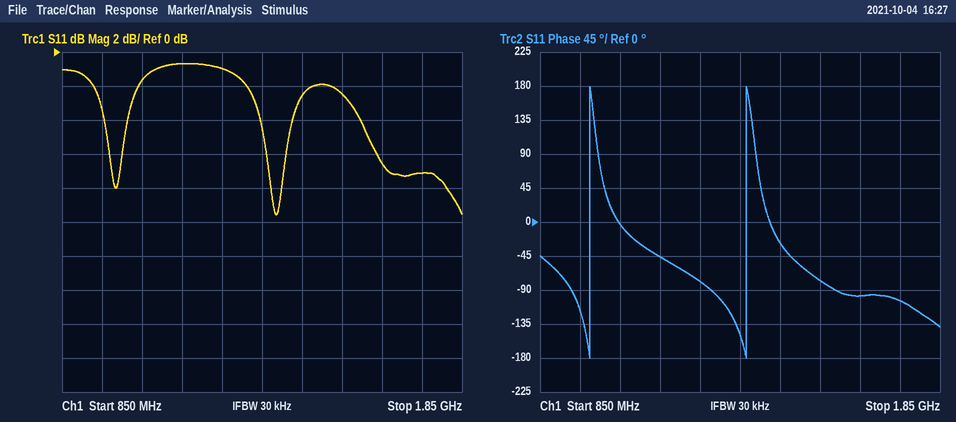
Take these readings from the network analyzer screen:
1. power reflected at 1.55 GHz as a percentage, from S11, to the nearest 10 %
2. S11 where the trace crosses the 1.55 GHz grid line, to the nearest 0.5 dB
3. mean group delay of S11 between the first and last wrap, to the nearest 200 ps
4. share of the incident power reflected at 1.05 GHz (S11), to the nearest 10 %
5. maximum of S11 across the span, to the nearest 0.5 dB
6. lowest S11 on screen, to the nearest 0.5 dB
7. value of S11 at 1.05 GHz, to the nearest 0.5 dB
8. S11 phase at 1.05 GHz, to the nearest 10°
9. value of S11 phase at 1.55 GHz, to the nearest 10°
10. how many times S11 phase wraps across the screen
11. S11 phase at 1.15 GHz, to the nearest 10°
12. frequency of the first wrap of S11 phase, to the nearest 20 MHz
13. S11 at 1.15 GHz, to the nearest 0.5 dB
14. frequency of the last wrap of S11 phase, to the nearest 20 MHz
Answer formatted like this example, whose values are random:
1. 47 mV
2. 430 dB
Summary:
1. 60 %
2. -2.5 dB
3. 2.6 ns
4. 70 %
5. -0.5 dB
6. -9.5 dB
7. -1.5 dB
8. 0°
9. -80°
10. 2
11. -50°
12. 980 MHz
13. -0.5 dB
14. 1.36 GHz
